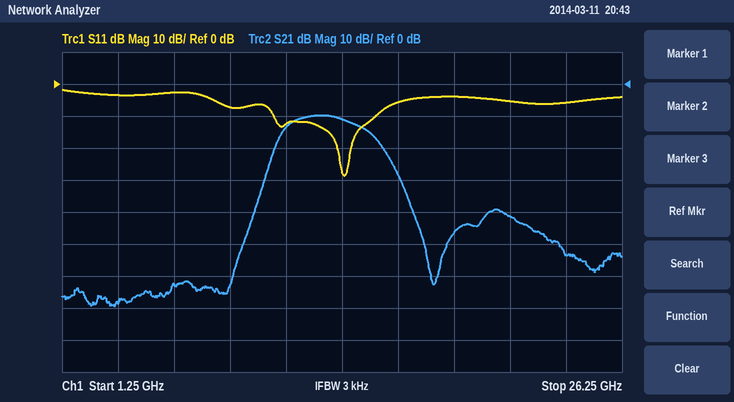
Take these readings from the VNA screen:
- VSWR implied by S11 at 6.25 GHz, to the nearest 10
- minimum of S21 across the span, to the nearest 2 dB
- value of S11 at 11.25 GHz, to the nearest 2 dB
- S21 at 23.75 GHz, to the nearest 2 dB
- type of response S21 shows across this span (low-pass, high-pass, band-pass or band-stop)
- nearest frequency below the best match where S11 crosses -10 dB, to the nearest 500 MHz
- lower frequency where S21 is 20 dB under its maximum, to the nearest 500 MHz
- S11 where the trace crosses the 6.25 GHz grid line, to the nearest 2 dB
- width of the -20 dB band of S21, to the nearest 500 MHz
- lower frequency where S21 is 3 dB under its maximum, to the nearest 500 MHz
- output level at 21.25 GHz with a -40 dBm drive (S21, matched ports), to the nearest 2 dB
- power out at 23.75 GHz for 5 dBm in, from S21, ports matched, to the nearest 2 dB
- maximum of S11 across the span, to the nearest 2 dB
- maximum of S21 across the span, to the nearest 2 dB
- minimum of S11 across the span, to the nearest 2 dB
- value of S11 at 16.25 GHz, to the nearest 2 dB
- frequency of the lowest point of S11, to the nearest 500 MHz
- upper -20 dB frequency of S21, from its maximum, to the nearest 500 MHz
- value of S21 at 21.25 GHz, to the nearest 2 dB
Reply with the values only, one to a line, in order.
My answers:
10
-70 dB
-12 dB
-54 dB
band-pass
10.5 GHz
10.5 GHz
-2 dB
6.0 GHz
11.5 GHz
-82 dBm
-48 dBm
-2 dB
-10 dB
-28 dB
-6 dB
14.0 GHz
16.5 GHz
-42 dB
